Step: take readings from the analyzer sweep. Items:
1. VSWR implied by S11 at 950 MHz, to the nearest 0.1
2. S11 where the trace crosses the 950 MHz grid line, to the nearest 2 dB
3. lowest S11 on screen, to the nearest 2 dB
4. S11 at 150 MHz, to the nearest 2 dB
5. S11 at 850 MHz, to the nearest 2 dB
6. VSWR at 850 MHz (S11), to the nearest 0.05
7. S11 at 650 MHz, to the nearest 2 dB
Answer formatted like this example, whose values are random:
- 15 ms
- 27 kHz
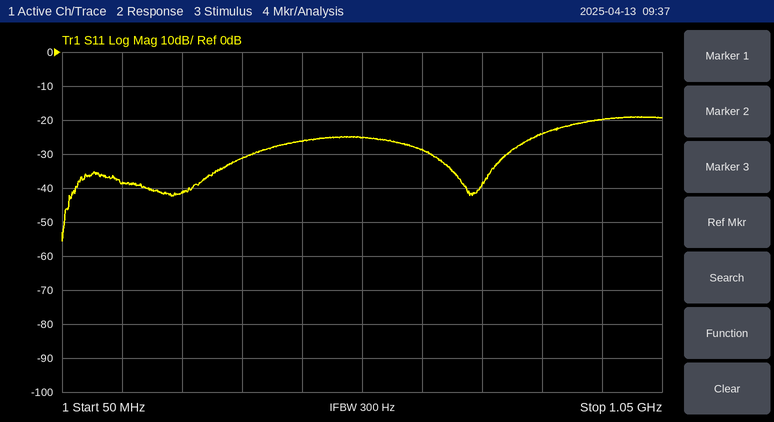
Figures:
- 1.2
- -20 dB
- -56 dB
- -38 dB
- -24 dB
- 1.15
- -28 dB
